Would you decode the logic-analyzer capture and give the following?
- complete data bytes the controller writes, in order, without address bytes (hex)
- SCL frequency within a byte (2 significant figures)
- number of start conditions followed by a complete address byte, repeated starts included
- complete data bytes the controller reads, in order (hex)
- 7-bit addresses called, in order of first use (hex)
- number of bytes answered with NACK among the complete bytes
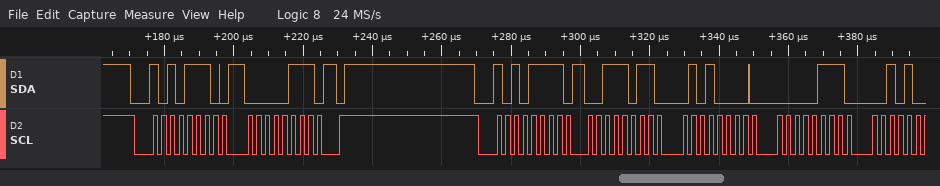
07
400 kHz
2
3B 50 07
0x57
0
